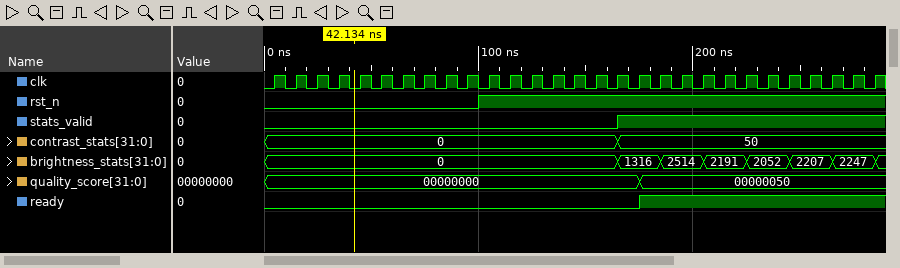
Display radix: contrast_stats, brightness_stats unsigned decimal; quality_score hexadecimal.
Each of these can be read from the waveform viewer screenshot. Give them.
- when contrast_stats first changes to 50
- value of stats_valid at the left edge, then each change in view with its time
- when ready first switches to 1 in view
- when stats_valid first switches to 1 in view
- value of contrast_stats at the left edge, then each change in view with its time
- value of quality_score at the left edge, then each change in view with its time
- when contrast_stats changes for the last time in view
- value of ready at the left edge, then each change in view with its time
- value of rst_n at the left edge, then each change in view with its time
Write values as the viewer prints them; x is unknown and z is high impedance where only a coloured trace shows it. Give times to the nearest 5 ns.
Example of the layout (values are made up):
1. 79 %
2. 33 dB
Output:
1. 165 ns
2. 0, 1 at 165 ns
3. 175 ns
4. 165 ns
5. 0, 50 at 165 ns
6. 00000000, 00000050 at 175 ns
7. 165 ns
8. 0, 1 at 175 ns
9. 0, 1 at 100 ns
